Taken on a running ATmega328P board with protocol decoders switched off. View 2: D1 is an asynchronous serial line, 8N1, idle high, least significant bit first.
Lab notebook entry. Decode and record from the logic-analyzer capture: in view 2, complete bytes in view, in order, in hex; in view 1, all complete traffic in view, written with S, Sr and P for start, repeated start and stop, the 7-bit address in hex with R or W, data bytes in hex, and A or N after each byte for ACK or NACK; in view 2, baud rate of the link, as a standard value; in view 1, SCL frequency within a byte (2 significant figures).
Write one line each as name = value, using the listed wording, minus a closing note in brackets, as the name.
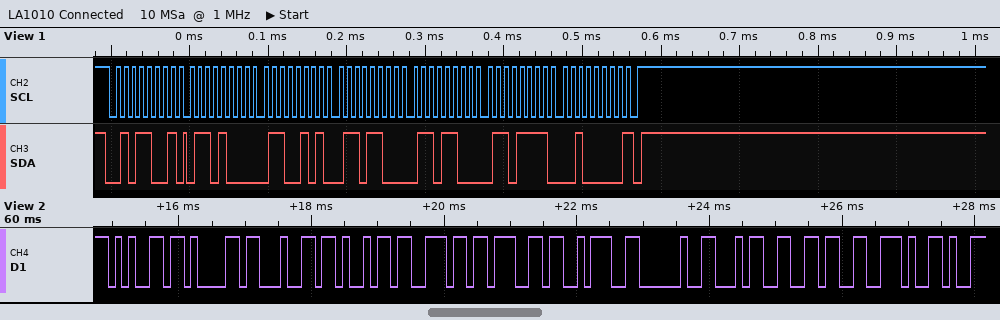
in view 2, complete bytes in view, in order, in hex = 65 61 64 69 6E 67 3A 20 34 36 2E
in view 1, all complete traffic in view, written with S, Sr and P for start, repeated start and stop, the 7-bit address in hex with R or W, data bytes in hex, and A or N after each byte for ACK or NACK = S 2CR A 68 A 65 A 6C A 6C A 6F A 20 N P
in view 2, baud rate of the link, as a standard value = 9600 baud
in view 1, SCL frequency within a byte = 100 kHz
